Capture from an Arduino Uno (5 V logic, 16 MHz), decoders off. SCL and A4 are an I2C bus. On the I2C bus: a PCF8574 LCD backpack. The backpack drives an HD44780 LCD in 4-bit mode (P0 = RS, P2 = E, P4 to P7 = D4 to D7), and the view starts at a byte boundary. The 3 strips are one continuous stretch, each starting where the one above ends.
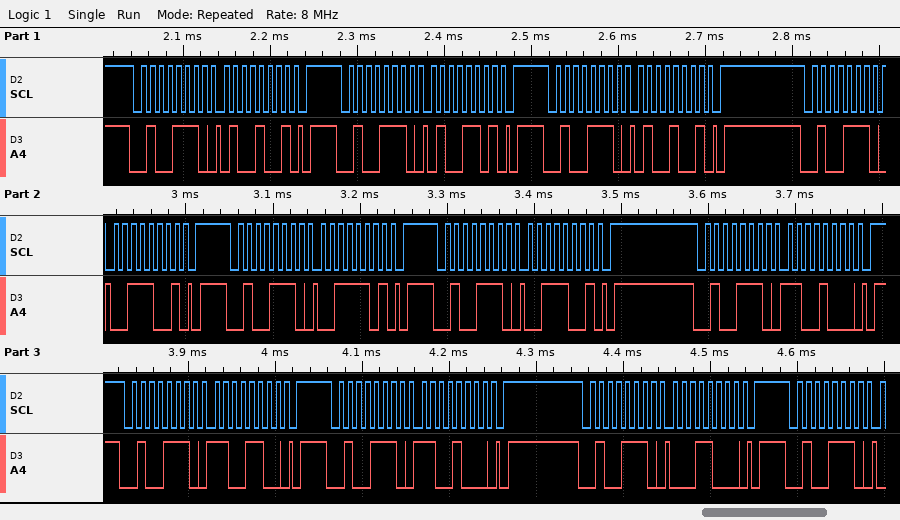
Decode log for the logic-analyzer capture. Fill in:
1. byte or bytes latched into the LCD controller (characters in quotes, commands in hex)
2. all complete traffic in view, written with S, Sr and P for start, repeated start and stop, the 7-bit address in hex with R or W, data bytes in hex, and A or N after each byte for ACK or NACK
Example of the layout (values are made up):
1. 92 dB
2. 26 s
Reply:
1. 'C'
2. S 27W A 49 A P S 27W A 4D A P S 27W A 49 A P S 27W A 39 A P S 27W A 3D A P S 27W A 39 A P S 27W A C8 A P S 27W A CC A P S 27W A C8 A P S 27W A 18 A P S 27W A
